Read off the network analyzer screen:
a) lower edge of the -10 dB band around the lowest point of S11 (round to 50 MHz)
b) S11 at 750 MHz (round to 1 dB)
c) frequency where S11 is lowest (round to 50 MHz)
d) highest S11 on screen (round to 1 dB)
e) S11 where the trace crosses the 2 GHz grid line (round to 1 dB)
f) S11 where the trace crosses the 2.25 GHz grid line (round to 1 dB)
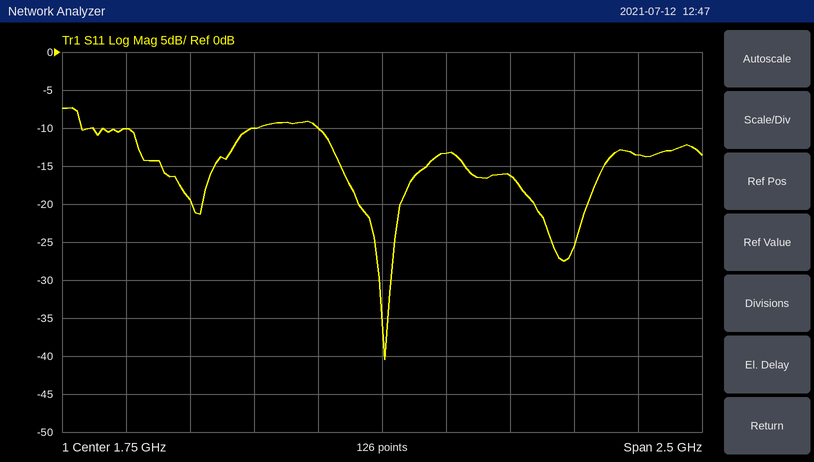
1.50 GHz
-10 dB
1.75 GHz
-7 dB
-13 dB
-16 dB
